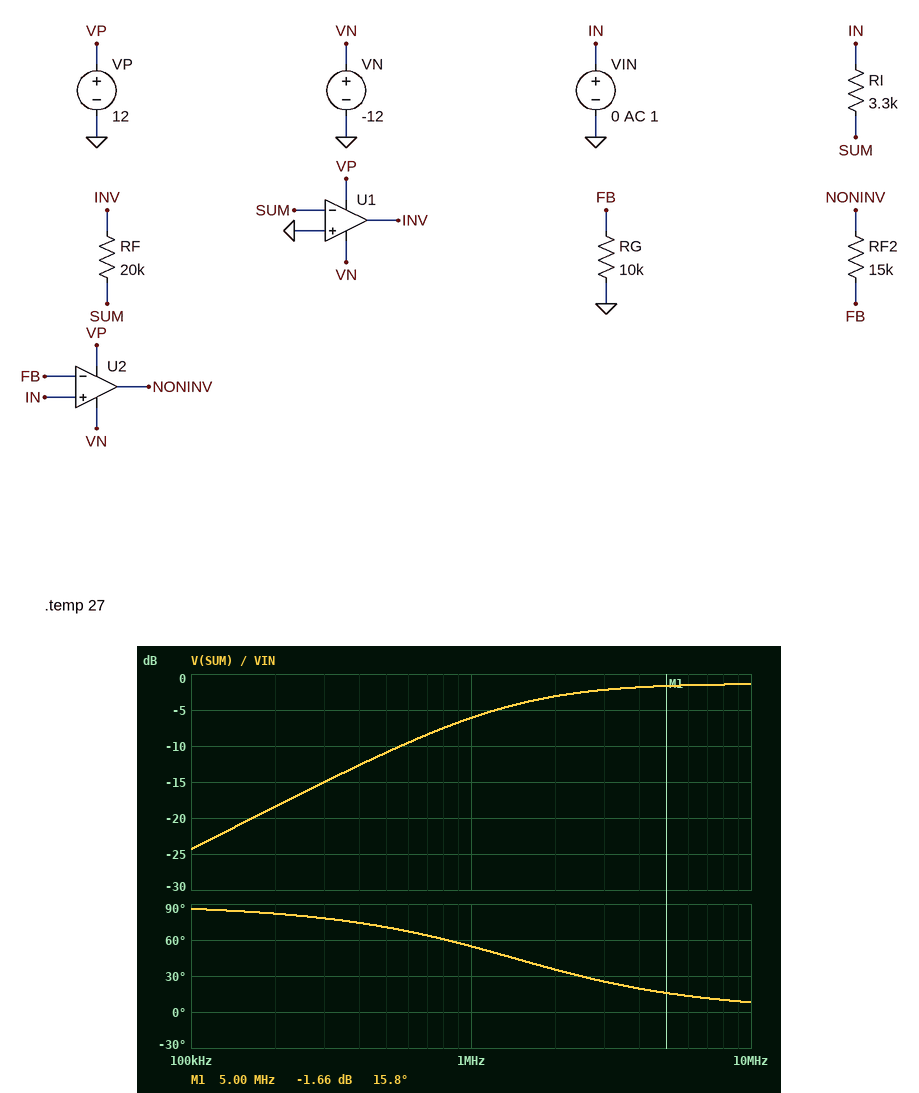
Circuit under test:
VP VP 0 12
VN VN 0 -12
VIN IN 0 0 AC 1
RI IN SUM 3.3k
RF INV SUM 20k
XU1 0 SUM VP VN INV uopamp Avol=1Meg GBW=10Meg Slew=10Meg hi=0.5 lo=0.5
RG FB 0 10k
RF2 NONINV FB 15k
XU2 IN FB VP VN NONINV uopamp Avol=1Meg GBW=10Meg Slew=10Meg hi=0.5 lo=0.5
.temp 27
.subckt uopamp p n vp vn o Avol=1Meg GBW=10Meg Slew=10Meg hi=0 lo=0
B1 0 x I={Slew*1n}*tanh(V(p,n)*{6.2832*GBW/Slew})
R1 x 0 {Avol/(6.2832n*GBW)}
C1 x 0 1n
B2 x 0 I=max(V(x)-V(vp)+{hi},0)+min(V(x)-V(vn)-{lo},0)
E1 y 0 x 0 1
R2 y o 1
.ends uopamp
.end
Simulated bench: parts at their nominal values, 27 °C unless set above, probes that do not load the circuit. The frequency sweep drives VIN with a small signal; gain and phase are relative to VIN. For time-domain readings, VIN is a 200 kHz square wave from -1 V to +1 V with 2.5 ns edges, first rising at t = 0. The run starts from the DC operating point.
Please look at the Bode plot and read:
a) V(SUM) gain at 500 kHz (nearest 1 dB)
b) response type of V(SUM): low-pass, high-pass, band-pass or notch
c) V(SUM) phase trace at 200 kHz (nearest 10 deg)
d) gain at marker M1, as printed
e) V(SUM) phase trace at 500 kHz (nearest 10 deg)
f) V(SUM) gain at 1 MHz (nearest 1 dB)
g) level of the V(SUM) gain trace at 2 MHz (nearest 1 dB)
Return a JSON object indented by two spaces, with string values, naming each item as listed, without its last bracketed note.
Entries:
{
  "V(SUM) gain at 500 kHz": "-11 dB",
  "response type of V(SUM): low-pass, high-pass, band-pass or notch": "high-pass",
  "V(SUM) phase trace at 200 kHz": "80 deg",
  "gain at marker M1, as printed": "-1.66 dB",
  "V(SUM) phase trace at 500 kHz": "70 deg",
  "V(SUM) gain at 1 MHz": "-6 dB",
  "level of the V(SUM) gain trace at 2 MHz": "-3 dB"
}
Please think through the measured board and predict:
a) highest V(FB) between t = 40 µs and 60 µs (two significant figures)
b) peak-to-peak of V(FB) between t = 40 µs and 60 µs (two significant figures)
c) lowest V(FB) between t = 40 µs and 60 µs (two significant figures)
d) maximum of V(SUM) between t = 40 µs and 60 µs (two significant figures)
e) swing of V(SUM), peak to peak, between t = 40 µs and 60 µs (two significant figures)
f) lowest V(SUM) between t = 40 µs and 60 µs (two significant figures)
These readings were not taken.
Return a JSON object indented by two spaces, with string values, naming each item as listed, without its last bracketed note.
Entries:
{
  "highest V(FB) between t = 40 µs and 60 µs": "1.0 V",
  "peak-to-peak of V(FB) between t = 40 µs and 60 µs": "2.0 V",
  "lowest V(FB) between t = 40 µs and 60 µs": "-1.0 V",
  "maximum of V(SUM) between t = 40 µs and 60 µs": "1.7 V",
  "swing of V(SUM), peak to peak, between t = 40 µs and 60 µs": "3.4 V",
  "lowest V(SUM) between t = 40 µs and 60 µs": "-1.7 V"
}
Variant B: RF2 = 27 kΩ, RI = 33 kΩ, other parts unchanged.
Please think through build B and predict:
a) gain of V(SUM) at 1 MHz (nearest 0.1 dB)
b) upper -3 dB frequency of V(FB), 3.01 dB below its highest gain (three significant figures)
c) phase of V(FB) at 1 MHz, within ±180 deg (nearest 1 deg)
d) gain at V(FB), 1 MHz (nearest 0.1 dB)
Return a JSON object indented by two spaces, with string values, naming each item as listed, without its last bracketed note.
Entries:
{
  "gain of V(SUM) at 1 MHz": "-24.5 dB",
  "upper -3 dB frequency of V(FB), 3.01 dB below its highest gain": "2.70 MHz",
  "phase of V(FB) at 1 MHz, within ±180 deg": "-20 deg",
  "gain at V(FB), 1 MHz": "-0.6 dB"
}
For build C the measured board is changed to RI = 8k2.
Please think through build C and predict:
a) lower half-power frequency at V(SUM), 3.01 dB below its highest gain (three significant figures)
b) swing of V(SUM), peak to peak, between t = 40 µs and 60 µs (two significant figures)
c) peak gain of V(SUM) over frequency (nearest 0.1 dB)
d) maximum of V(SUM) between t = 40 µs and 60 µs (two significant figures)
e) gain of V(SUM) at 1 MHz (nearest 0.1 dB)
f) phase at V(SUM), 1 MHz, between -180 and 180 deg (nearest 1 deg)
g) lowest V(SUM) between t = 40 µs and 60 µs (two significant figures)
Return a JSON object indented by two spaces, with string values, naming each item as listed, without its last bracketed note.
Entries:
{
  "lower half-power frequency at V(SUM), 3.01 dB below its highest gain": "2.91 MHz",
  "swing of V(SUM), peak to peak, between t = 40 µs and 60 µs": "2.8 V",
  "peak gain of V(SUM) over frequency": "-3.0 dB",
  "maximum of V(SUM) between t = 40 µs and 60 µs": "1.4 V",
  "gain of V(SUM) at 1 MHz": "-12.7 dB",
  "phase at V(SUM), 1 MHz, between -180 and 180 deg": "71 deg",
  "lowest V(SUM) between t = 40 µs and 60 µs": "-1.4 V"
}
